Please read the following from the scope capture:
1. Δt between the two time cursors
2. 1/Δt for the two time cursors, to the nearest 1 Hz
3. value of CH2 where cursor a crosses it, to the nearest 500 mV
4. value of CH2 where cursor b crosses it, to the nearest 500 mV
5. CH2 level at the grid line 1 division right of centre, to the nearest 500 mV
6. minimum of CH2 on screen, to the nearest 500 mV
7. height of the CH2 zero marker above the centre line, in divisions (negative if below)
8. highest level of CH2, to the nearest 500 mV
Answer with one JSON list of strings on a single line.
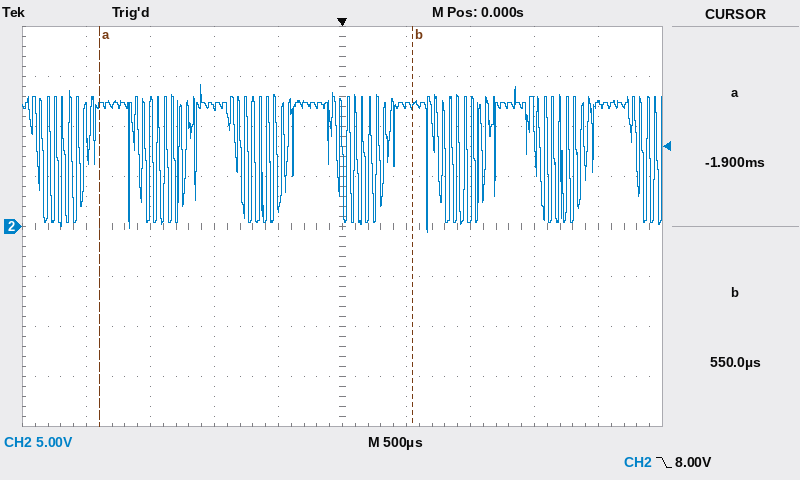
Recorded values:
["2.45 ms", "408 Hz", "12.0 V", "12.0 V", "12.0 V", "-500 mV", "0.0 div", "14.0 V"]
